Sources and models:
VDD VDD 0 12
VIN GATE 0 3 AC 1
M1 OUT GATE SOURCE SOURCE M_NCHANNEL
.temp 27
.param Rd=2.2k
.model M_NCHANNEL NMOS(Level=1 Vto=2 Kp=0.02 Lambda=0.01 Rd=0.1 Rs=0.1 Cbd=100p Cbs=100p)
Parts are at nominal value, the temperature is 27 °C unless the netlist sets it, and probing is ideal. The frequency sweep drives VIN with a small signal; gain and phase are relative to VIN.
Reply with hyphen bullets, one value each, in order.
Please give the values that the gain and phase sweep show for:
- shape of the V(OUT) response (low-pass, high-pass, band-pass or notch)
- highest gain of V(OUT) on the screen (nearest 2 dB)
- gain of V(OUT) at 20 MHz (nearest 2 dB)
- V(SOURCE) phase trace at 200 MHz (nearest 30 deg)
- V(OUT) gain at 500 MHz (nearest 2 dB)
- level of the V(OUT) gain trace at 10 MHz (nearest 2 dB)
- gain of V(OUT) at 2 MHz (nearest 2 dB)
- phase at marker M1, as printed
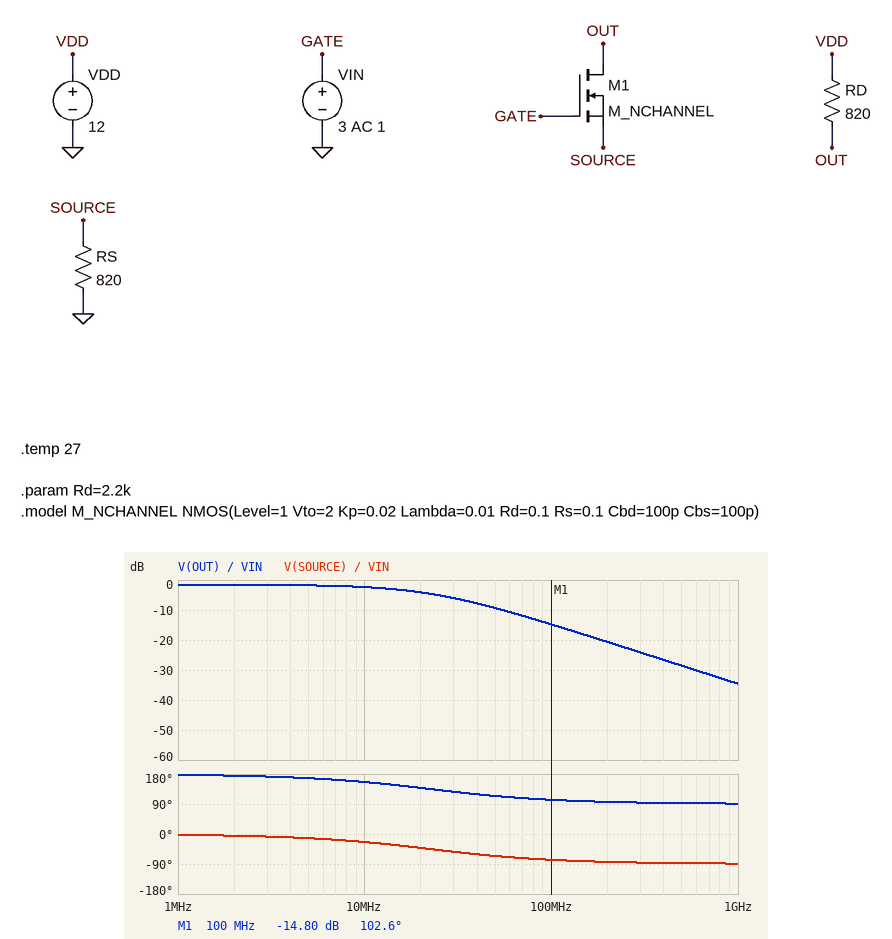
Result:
- low-pass
- -2 dB
- -4 dB
- -90 deg
- -28 dB
- -2 dB
- -2 dB
- 102.6 deg
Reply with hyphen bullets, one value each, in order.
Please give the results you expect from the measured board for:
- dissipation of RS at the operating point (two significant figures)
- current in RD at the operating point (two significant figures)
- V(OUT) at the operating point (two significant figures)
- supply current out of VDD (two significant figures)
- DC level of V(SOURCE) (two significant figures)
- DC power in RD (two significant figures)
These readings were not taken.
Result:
- 630 µW
- 880 µA
- 11 V
- 880 µA
- 720 mV
- 630 µW
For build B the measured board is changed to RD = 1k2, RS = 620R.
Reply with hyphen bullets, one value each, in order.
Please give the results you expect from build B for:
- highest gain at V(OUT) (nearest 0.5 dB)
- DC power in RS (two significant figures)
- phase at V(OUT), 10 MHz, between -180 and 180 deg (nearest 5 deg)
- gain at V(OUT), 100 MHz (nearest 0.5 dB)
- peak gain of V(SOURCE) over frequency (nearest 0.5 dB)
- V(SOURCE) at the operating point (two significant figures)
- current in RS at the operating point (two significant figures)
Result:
- 4.0 dB
- 750 µW
- 150 deg
- -11.5 dB
- -2.0 dB
- 680 mV
- 1.1 mA
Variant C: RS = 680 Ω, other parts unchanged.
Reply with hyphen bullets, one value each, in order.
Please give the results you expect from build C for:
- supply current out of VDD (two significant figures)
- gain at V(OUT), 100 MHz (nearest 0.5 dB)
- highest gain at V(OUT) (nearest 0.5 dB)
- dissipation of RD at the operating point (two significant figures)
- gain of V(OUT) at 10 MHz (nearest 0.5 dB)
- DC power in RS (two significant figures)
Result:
- 1.0 mA
- -13.5 dB
- 0 dB
- 860 µW
- -1.0 dB
- 710 µW
